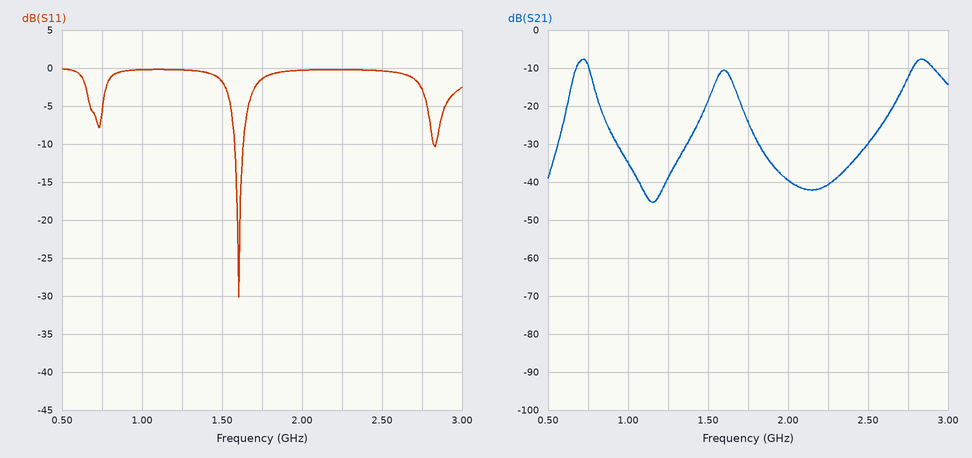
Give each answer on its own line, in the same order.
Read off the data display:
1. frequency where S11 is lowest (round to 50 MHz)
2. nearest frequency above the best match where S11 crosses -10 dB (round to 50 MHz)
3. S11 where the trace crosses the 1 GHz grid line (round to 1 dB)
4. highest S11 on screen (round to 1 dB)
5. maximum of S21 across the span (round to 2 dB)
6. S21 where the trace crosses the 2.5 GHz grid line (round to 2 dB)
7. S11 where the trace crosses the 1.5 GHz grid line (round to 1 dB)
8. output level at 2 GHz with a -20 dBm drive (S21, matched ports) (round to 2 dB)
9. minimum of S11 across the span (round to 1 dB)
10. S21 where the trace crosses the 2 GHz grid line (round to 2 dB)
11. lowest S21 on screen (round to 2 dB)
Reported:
1.60 GHz
1.65 GHz
0 dB
0 dB
-8 dB
-30 dB
-2 dB
-60 dBm
-30 dB
-40 dB
-46 dB
